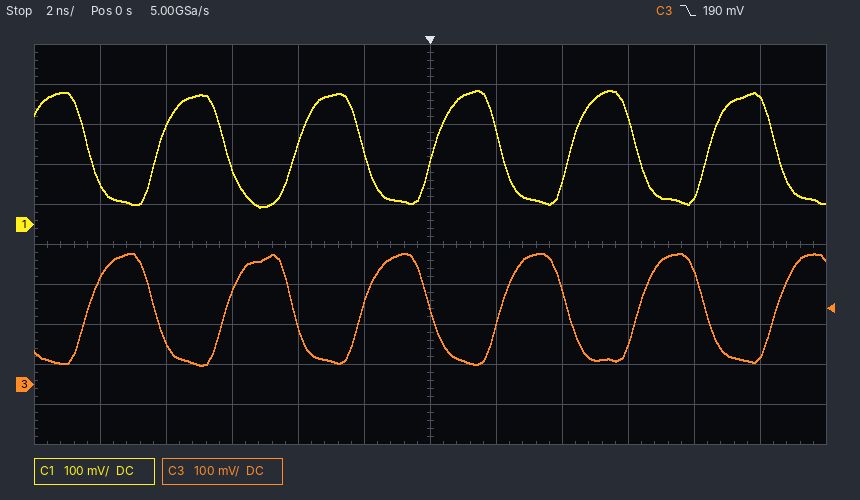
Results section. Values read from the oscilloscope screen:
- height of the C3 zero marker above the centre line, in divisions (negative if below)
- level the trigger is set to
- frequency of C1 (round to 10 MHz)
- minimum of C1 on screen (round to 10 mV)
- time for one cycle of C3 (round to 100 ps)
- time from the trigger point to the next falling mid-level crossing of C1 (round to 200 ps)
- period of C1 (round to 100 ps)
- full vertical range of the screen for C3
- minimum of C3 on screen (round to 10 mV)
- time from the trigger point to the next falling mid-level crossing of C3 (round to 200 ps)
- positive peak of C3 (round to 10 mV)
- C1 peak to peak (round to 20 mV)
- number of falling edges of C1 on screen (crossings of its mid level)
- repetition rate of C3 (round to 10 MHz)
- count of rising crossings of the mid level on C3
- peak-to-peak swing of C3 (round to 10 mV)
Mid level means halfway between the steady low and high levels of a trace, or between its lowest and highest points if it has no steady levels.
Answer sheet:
-3.5 div
190 mV
240 MHz
40 mV
4.2 ns
2.2 ns
4.2 ns
1 V
50 mV
4.2 ns
330 mV
300 mV
6
240 MHz
6
280 mV
